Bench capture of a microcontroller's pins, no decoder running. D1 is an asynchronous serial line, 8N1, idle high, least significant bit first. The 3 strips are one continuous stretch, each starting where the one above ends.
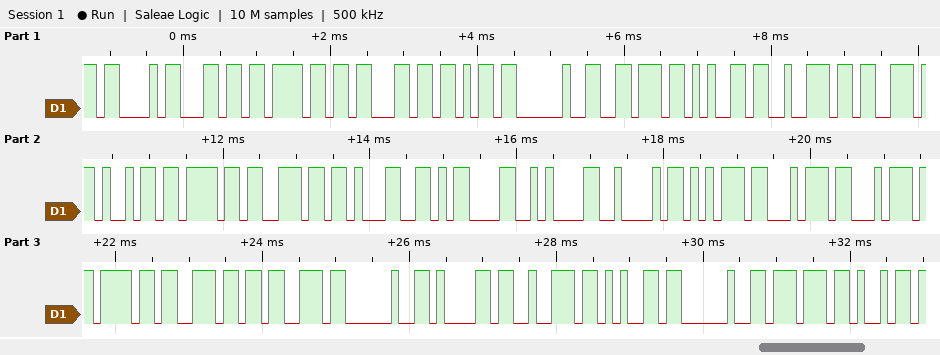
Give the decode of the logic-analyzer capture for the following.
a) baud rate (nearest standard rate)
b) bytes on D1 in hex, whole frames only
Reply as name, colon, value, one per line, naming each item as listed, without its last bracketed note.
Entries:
baud rate: 9600 baud
bytes on D1 in hex, whole frames only: 43 6C 6F 63 6B 20 76 65 72 73 69 6F 6E 31 0D 0A 42 75 74 74 6F 6E 73 20 61 72 65 20 77 69
